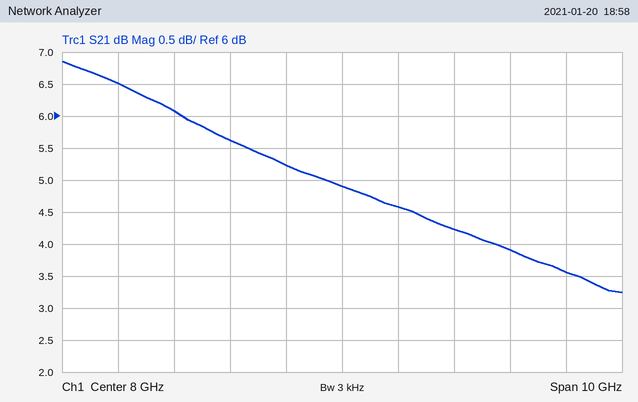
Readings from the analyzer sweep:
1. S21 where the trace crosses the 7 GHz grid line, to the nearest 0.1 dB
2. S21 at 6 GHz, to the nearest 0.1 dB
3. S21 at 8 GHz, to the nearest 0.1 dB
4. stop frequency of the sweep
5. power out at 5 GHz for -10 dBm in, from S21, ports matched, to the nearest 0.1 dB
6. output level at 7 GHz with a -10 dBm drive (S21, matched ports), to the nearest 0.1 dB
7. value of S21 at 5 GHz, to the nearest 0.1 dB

5.2 dB
5.6 dB
4.9 dB
13 GHz
-3.9 dBm
-4.8 dBm
6.1 dB
